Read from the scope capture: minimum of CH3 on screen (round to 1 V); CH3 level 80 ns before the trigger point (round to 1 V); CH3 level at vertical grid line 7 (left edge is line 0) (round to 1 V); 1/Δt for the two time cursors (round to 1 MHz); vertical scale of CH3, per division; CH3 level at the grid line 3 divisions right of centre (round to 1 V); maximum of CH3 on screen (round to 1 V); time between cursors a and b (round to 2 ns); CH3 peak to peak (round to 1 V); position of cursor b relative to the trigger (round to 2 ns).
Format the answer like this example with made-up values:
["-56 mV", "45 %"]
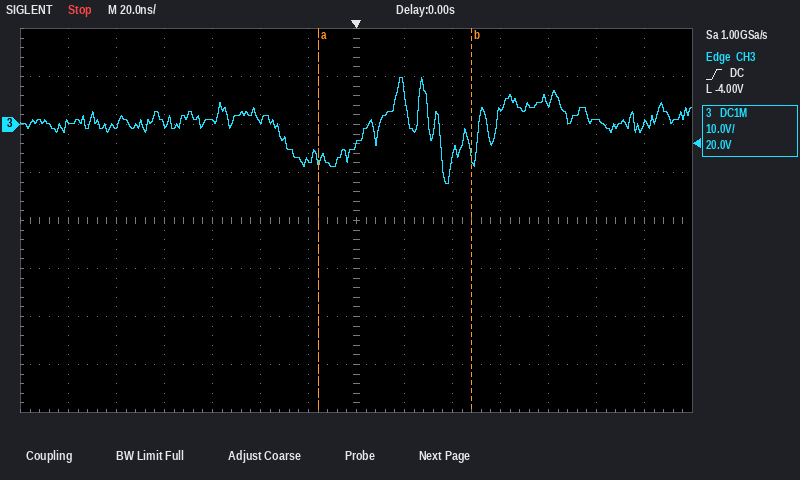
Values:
["-12 V", "0 V", "-4 V", "16 MHz", "10 V", "3 V", "10 V", "64 ns", "22 V", "+48 ns"]
